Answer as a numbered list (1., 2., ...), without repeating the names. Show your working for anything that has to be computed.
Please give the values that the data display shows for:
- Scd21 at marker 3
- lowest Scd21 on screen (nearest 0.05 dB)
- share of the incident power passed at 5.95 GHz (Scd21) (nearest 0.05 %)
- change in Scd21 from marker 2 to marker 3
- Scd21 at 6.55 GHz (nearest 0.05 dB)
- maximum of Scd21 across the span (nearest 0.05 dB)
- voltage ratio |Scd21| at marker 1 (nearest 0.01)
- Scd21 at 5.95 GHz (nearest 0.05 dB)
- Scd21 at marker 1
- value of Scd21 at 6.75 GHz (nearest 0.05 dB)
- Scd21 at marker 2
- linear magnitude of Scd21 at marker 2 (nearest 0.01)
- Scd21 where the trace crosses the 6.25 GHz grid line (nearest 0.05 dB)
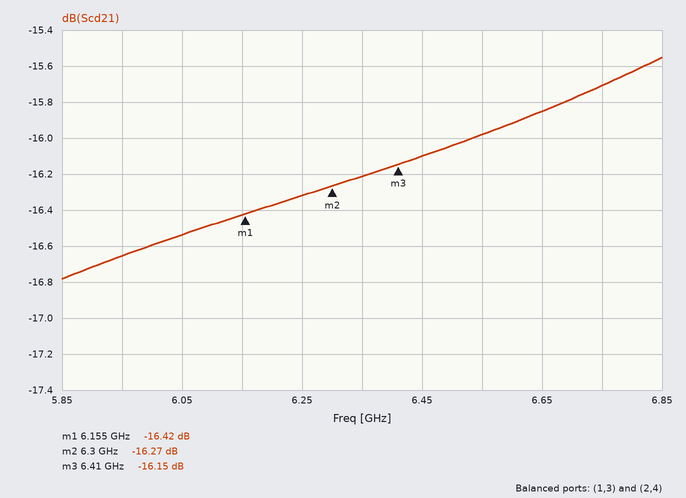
1. -16.15 dB
2. -16.80 dB
3. 10^(-16.65/10) ≈ 2.16 %, so 2.15 % to the nearest 0.05 %
4. -16.15 − (-16.27) = 0.12 dB
5. -16.00 dB
6. -15.55 dB
7. 10^(-16.42/20) ≈ 0.15
8. -16.65 dB
9. -16.42 dB
10. -15.70 dB
11. -16.27 dB
12. 10^(-16.27/20) ≈ 0.15
13. -16.30 dB
